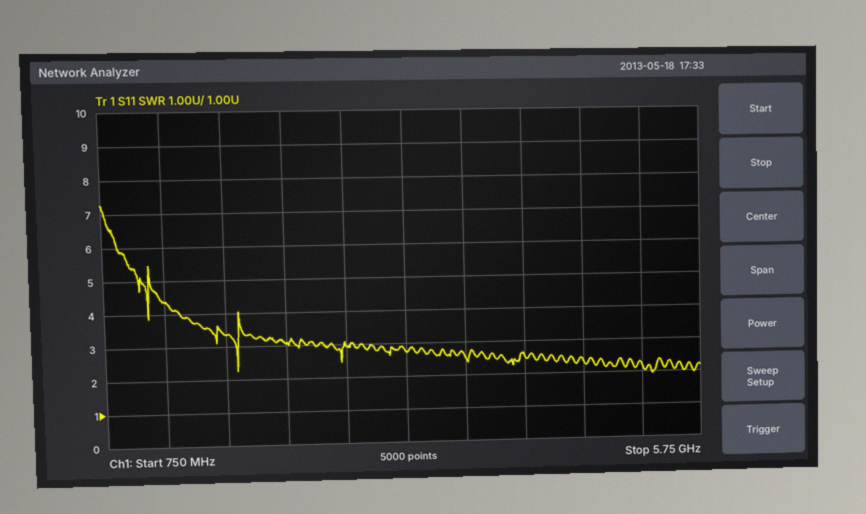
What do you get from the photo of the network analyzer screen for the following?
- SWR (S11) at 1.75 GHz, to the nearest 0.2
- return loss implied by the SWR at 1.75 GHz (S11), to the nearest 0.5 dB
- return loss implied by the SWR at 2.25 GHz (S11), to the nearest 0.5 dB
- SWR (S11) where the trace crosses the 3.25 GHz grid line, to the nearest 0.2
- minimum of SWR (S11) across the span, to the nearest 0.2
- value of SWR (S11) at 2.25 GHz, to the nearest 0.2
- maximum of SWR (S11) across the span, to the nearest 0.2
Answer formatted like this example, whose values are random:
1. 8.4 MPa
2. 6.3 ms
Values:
1. 3.4
2. 5.5 dB
3. 6.0 dB
4. 2.8
5. 2.0
6. 3.0
7. 7.2
